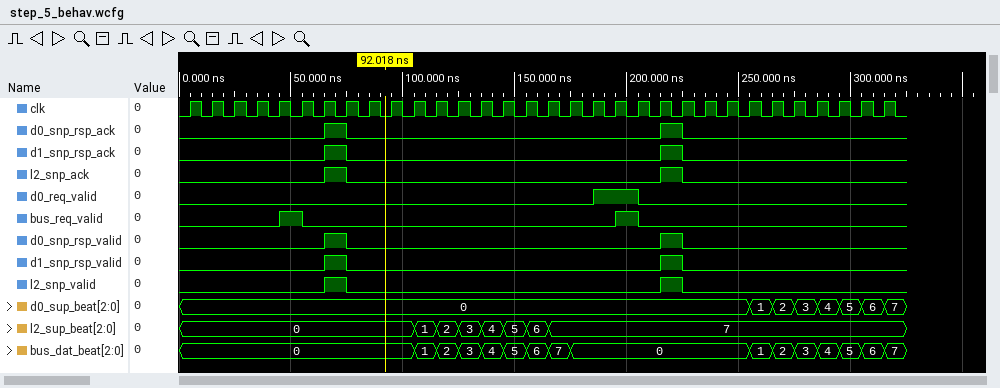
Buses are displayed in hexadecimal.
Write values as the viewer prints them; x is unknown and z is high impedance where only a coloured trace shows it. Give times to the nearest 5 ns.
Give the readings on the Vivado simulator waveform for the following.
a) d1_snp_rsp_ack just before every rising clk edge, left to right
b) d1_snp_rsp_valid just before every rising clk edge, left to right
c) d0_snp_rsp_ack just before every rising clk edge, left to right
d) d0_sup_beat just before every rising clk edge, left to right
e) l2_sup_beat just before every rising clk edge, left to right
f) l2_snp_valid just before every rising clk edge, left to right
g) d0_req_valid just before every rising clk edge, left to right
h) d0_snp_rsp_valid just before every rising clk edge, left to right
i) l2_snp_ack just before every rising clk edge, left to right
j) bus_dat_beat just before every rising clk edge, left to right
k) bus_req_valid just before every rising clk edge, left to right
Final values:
0 0 0 0 0 0 0 1 0 0 0 0 0 0 0 0 0 0 0 0 0 0 1 0 0 0 0 0 0 0 0 0
0 0 0 0 0 0 0 1 0 0 0 0 0 0 0 0 0 0 0 0 0 0 1 0 0 0 0 0 0 0 0 0
0 0 0 0 0 0 0 1 0 0 0 0 0 0 0 0 0 0 0 0 0 0 1 0 0 0 0 0 0 0 0 0
0, 0, 0, 0, 0, 0, 0, 0, 0, 0, 0, 0, 0, 0, 0, 0, 0, 0, 0, 0, 0, 0, 0, 0, 0, 0, 1, 2, 3, 4, 5, 6
0, 0, 0, 0, 0, 0, 0, 0, 0, 0, 0, 1, 2, 3, 4, 5, 6, 7, 7, 7, 7, 7, 7, 7, 7, 7, 7, 7, 7, 7, 7, 7
0 0 0 0 0 0 0 1 0 0 0 0 0 0 0 0 0 0 0 0 0 0 1 0 0 0 0 0 0 0 0 0
0 0 0 0 0 0 0 0 0 0 0 0 0 0 0 0 0 0 0 1 1 0 0 0 0 0 0 0 0 0 0 0
0 0 0 0 0 0 0 1 0 0 0 0 0 0 0 0 0 0 0 0 0 0 1 0 0 0 0 0 0 0 0 0
0 0 0 0 0 0 0 1 0 0 0 0 0 0 0 0 0 0 0 0 0 0 1 0 0 0 0 0 0 0 0 0
0, 0, 0, 0, 0, 0, 0, 0, 0, 0, 0, 1, 2, 3, 4, 5, 6, 7, 0, 0, 0, 0, 0, 0, 0, 0, 1, 2, 3, 4, 5, 6
0 0 0 0 0 1 0 0 0 0 0 0 0 0 0 0 0 0 0 0 1 0 0 0 0 0 0 0 0 0 0 0
